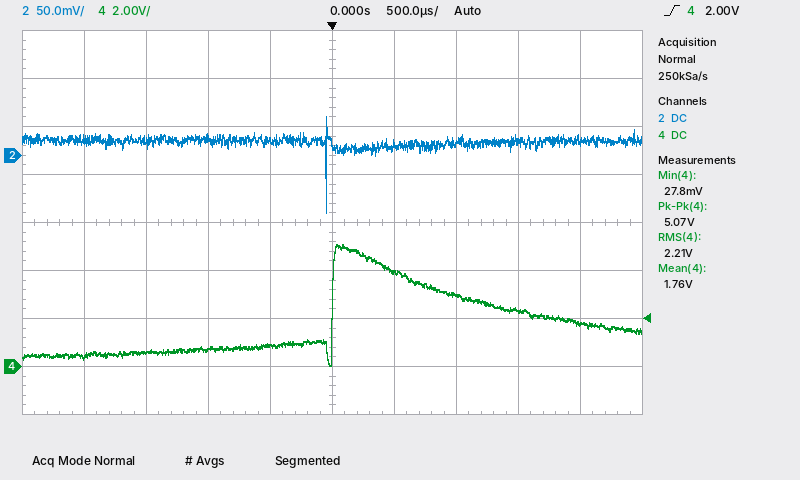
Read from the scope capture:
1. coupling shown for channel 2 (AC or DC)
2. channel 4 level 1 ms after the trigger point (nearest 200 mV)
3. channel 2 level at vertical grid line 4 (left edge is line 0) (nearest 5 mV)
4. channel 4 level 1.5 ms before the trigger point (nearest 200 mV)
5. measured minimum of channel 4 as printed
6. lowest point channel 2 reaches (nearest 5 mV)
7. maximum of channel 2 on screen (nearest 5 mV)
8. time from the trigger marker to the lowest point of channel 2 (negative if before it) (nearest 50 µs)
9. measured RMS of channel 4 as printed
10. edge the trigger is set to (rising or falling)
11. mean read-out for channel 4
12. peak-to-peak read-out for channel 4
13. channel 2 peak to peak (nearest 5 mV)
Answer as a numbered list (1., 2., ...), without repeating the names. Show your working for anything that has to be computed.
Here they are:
1. DC
2. 3.0 V
3. 15 mV
4. 600 mV
5. 27.8 mV
6. -60 mV
7. 40 mV
8. -50 µs
9. 2.21 V
10. rising
11. 1.76 V
12. 5.07 V
13. 40 mV − (-60 mV) = 100 mV
